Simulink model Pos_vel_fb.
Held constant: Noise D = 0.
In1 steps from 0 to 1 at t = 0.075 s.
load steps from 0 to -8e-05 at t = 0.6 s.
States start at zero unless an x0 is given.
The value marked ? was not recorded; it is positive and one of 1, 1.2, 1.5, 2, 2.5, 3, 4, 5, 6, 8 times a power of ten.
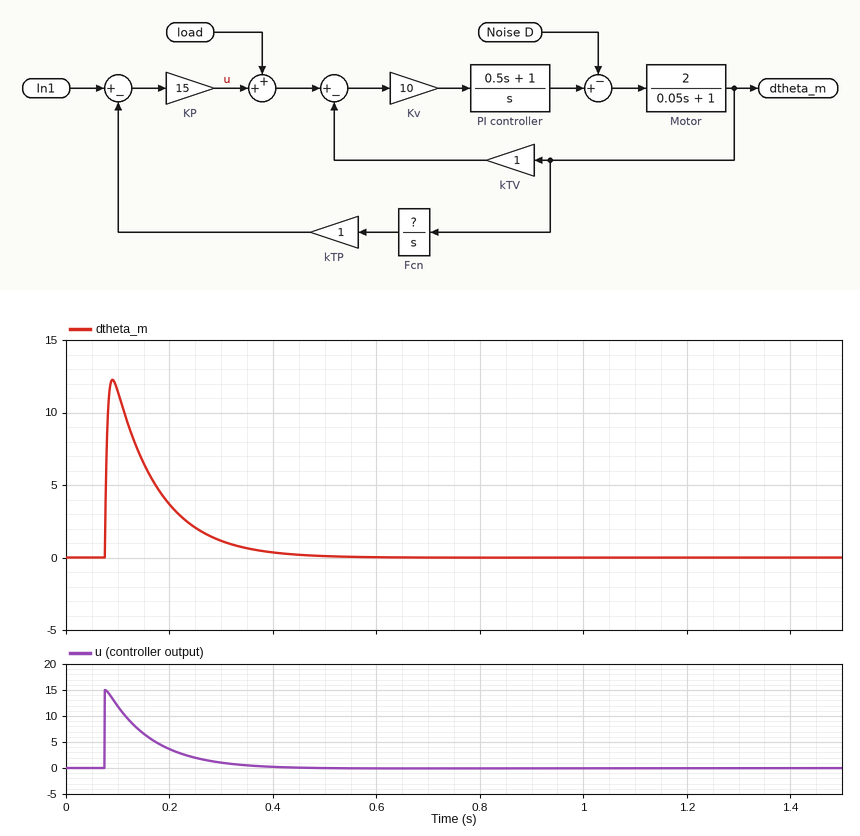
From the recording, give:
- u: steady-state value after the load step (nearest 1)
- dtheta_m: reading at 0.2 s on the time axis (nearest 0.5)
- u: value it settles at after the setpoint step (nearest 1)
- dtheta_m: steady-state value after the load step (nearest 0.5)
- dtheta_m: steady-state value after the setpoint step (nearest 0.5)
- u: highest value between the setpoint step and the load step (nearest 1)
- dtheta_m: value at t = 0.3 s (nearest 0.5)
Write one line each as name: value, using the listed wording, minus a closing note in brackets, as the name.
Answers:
u: steady-state value after the load step: 0
dtheta_m: reading at 0.2 s on the time axis: 3.5
u: value it settles at after the setpoint step: 0
dtheta_m: steady-state value after the load step: 0.0
dtheta_m: steady-state value after the setpoint step: 0.0
u: highest value between the setpoint step and the load step: 15
dtheta_m: value at t = 0.3 s: 1.0
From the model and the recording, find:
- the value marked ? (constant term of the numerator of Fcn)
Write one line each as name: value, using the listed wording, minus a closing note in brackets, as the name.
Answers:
the value marked ?: 0.8
